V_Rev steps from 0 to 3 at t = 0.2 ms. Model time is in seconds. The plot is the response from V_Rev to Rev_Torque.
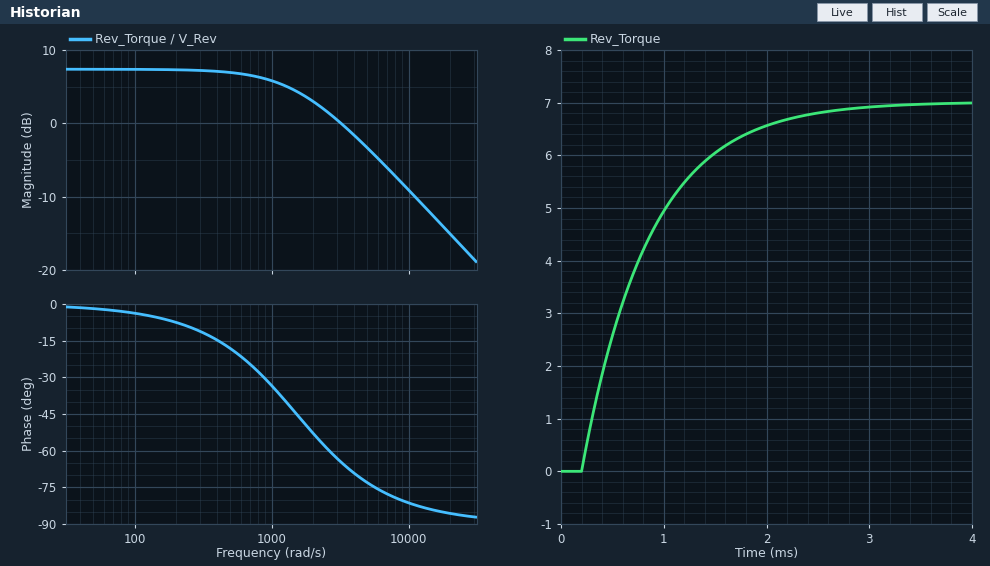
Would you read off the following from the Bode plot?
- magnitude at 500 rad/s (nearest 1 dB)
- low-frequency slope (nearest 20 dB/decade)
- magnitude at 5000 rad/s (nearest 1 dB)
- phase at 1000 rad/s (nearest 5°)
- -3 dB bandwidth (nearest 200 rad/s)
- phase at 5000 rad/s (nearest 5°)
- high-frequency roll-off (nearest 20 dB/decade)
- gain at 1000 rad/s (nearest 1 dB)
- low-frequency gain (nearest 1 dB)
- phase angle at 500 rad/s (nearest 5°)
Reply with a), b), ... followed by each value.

a) 7 dB
b) 0 dB/decade
c) -3 dB
d) -35°
e) 1600 rad/s
f) -75°
g) -20 dB/decade
h) 6 dB
i) 7 dB
j) -20°
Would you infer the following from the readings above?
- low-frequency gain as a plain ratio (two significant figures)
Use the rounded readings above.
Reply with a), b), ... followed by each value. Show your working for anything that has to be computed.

a) 10^(7 / 20) = 2.2
